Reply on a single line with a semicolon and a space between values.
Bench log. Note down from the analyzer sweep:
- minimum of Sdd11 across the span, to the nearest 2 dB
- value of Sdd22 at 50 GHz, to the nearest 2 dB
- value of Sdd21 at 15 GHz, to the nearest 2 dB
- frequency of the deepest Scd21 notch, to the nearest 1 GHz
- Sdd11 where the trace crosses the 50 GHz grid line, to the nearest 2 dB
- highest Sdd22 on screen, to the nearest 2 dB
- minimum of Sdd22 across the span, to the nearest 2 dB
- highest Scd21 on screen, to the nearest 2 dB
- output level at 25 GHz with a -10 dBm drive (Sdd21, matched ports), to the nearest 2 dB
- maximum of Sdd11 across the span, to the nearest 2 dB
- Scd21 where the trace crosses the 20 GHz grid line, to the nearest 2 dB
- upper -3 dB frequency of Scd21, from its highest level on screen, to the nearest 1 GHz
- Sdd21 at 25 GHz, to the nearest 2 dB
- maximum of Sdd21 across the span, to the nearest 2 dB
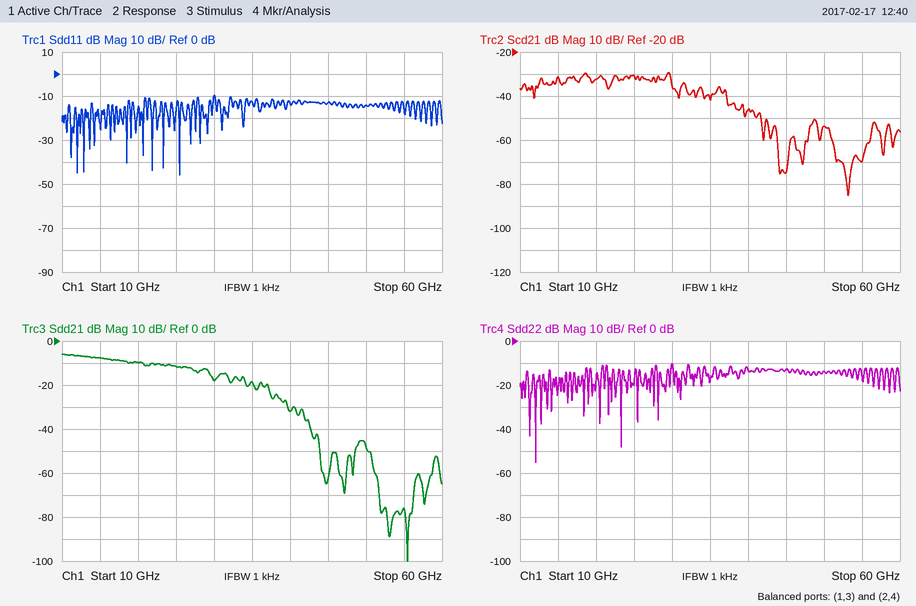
-46 dB; -14 dB; -8 dB; 53 GHz; -14 dB; -10 dB; -56 dB; -30 dB; -22 dBm; -10 dB; -32 dB; 30 GHz; -12 dB; -6 dB
